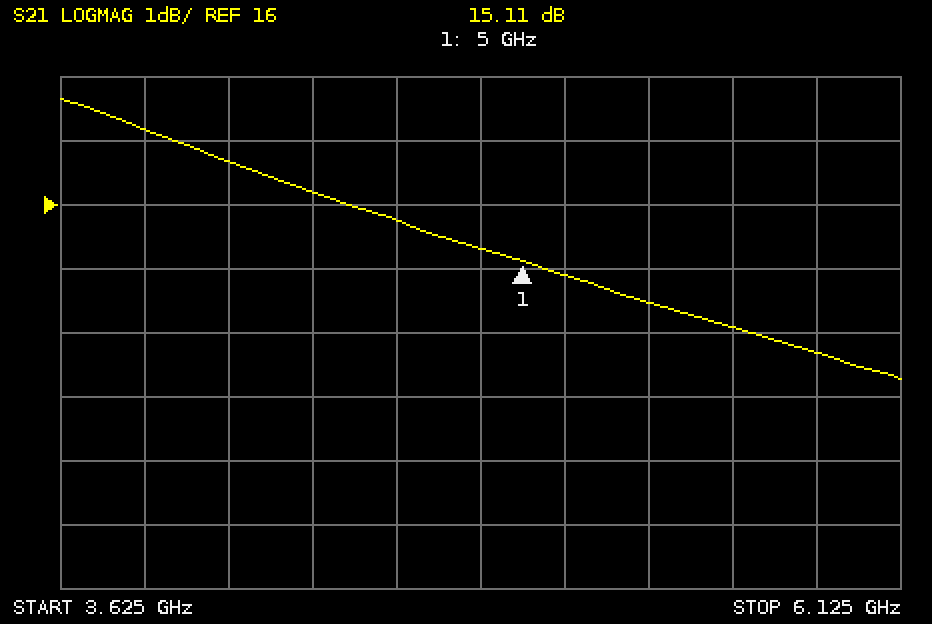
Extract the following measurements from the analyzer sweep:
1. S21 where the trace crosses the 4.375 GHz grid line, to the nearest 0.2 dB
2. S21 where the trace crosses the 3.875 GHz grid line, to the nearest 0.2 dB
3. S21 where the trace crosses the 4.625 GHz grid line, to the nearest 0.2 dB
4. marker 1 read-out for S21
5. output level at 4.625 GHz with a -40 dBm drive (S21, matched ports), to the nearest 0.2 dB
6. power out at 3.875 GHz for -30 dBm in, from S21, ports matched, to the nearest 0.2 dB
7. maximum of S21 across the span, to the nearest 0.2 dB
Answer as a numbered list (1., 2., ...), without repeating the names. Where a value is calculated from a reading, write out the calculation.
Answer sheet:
1. 16.2 dB
2. 17.2 dB
3. 15.8 dB
4. 15.11 dB
5. -40 dBm + (15.8 dB) = -24.2 dBm
6. -30 dBm + (17.2 dB) = -12.8 dBm
7. 17.6 dB
